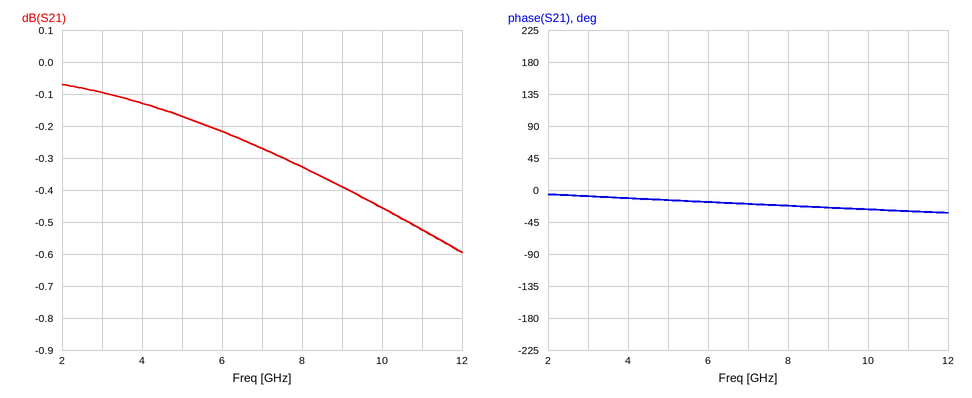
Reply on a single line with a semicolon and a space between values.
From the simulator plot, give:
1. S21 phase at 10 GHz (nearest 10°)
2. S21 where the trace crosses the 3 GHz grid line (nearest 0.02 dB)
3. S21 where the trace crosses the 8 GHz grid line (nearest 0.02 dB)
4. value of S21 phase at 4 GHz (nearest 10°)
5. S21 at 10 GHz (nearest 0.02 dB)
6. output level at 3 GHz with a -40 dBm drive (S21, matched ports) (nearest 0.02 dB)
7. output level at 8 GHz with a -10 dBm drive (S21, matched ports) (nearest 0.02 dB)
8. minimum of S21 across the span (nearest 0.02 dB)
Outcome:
-30°; -0.10 dB; -0.32 dB; -10°; -0.46 dB; -40.10 dBm; -10.32 dBm; -0.60 dB
